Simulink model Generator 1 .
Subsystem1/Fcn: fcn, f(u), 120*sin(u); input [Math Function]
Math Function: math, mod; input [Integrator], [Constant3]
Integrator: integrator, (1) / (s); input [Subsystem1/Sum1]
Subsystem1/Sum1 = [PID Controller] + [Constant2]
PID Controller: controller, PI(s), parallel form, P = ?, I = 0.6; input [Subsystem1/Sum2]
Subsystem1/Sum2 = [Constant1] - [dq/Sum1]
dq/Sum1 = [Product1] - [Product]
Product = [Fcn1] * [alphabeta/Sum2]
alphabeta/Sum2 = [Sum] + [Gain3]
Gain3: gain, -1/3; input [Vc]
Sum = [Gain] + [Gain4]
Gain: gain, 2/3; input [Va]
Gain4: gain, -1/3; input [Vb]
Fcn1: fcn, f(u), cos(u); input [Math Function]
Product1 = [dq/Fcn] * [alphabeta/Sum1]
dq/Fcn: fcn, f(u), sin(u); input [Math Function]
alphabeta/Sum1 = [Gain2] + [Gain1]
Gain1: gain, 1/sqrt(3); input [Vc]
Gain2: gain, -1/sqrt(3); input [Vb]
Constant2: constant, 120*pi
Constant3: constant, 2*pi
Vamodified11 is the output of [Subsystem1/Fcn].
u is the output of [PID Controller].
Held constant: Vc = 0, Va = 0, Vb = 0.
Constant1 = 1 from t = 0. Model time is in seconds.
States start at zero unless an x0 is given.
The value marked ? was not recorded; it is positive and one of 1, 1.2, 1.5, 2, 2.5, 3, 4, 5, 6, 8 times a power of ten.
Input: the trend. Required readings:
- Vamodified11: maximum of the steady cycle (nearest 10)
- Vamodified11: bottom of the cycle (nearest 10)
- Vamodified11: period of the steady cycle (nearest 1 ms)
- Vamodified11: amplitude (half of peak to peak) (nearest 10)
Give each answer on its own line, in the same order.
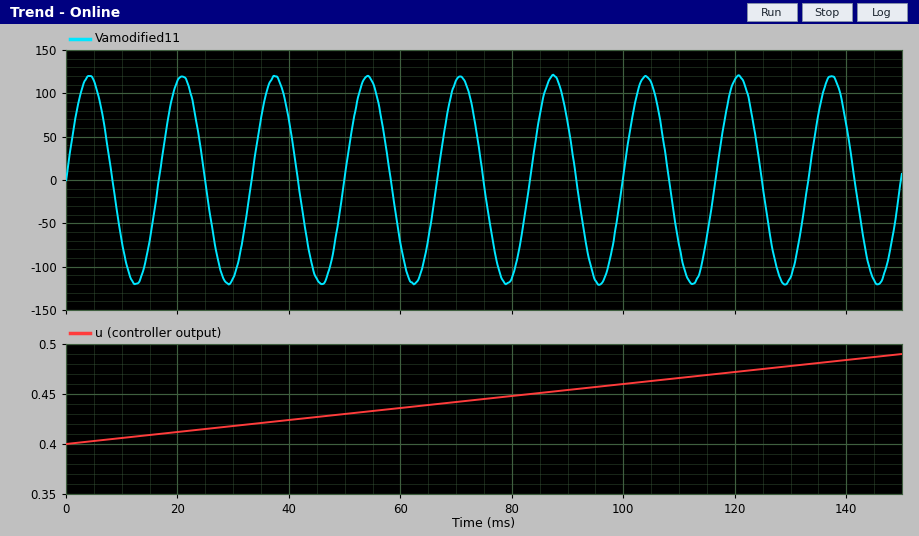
120
-120
17 ms
120
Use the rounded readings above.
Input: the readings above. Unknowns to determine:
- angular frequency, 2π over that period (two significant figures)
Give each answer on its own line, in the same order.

0.37 rad/ms
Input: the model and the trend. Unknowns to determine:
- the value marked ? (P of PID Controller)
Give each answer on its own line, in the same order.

0.4
